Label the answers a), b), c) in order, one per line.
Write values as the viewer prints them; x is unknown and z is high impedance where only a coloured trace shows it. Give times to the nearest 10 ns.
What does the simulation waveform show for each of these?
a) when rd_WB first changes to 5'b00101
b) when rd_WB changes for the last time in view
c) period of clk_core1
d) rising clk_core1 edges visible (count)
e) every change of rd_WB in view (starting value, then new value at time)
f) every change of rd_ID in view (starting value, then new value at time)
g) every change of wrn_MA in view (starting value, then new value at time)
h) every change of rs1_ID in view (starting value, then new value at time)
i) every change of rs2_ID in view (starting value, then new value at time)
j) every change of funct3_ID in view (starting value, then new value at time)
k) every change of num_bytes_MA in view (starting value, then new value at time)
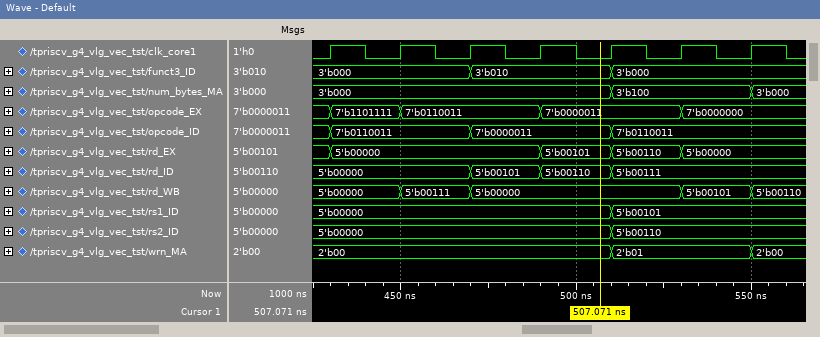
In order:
a) 530 ns
b) 550 ns
c) 20 ns
d) 7
e) 5'b00000, 5'b00111 at 450 ns, 5'b00000 at 470 ns, 5'b00101 at 530 ns, 5'b00110 at 550 ns
f) 5'b00000, 5'b00101 at 470 ns, 5'b00110 at 490 ns, 5'b00111 at 510 ns
g) 2'b00, 2'b01 at 510 ns, 2'b00 at 550 ns
h) 5'b00000, 5'b00101 at 510 ns
i) 5'b00000, 5'b00110 at 510 ns
j) 3'b000, 3'b010 at 470 ns, 3'b000 at 510 ns
k) 3'b000, 3'b100 at 510 ns, 3'b000 at 550 ns
